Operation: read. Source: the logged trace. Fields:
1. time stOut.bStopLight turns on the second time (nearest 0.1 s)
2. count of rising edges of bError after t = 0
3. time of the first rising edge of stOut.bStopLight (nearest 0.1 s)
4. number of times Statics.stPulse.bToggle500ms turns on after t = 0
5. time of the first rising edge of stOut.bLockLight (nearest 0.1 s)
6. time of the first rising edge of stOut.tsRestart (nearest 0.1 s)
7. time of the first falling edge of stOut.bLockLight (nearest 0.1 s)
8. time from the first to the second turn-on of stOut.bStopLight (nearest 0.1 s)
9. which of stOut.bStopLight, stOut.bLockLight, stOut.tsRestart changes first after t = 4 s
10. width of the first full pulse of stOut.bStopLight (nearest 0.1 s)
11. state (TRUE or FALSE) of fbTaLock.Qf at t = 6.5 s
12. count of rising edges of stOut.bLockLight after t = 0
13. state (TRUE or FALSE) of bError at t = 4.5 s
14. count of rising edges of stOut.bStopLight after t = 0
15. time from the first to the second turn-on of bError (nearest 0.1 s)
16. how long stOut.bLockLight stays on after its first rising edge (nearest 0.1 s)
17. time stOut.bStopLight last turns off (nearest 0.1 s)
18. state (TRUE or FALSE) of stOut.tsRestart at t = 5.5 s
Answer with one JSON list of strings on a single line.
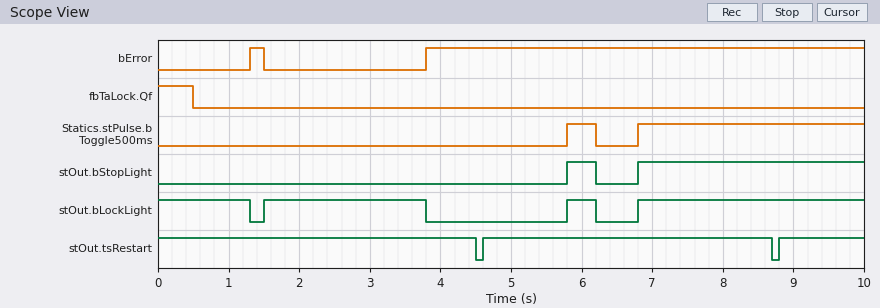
["6.8 s", "2", "5.8 s", "2", "1.5 s", "4.6 s", "1.3 s", "1.0 s", "stOut.tsRestart", "0.4 s", "FALSE", "3", "TRUE", "2", "2.5 s", "2.3 s", "6.2 s", "TRUE"]
